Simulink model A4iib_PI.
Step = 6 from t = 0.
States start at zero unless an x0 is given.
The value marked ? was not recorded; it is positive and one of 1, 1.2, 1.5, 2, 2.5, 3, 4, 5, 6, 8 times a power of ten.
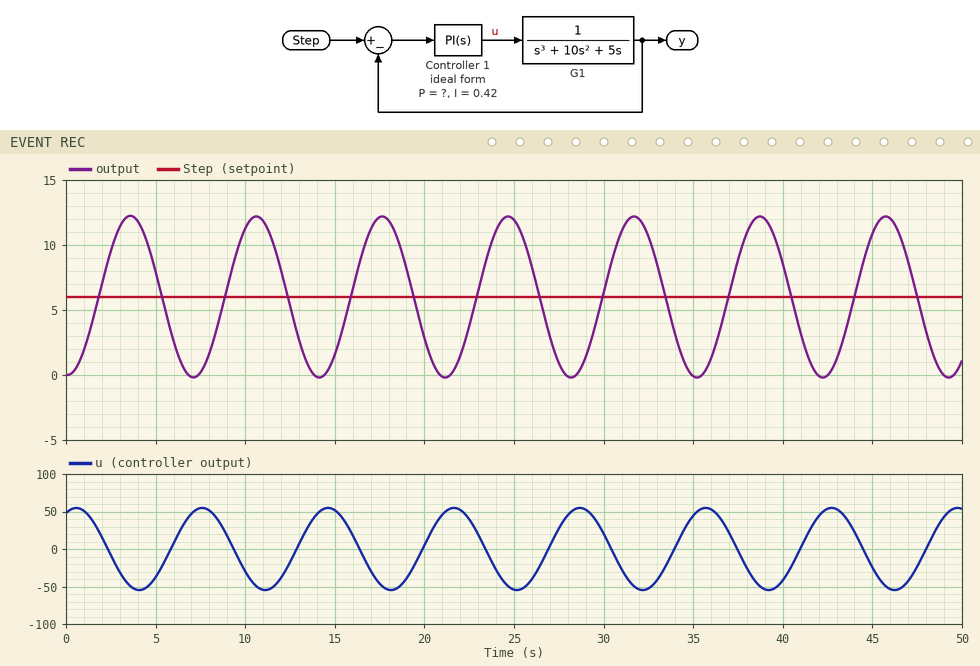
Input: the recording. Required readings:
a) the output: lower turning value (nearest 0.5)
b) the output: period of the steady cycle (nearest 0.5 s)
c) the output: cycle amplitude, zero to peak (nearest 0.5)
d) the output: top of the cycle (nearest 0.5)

0.0
7.0 s
6.0
12.0
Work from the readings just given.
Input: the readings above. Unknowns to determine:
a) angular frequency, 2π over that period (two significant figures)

0.90 rad/s
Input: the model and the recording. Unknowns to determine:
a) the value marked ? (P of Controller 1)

8
